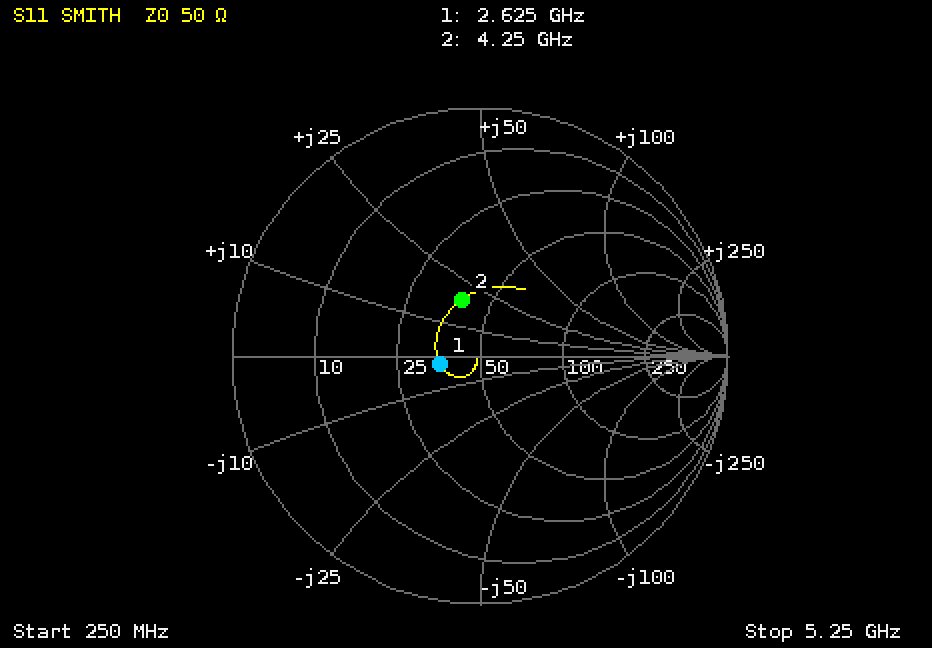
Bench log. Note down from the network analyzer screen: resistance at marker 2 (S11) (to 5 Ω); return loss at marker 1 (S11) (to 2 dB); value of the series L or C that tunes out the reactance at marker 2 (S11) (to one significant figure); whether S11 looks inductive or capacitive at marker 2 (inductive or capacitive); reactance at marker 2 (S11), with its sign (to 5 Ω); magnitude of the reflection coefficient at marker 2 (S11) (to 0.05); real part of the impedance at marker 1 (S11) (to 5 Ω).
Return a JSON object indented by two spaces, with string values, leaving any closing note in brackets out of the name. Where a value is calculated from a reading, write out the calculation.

{
  "resistance at marker 2 (S11)": "40 Ω",
  "return loss at marker 1 (S11)": "16 dB",
  "value of the series L or C that tunes out the reactance at marker 2 (S11)": "C = 1/(2π × 4.25 GHz × 20 Ω) ≈ 2 pF",
  "whether S11 looks inductive or capacitive at marker 2": "inductive",
  "reactance at marker 2 (S11), with its sign": "+20 Ω",
  "magnitude of the reflection coefficient at marker 2 (S11)": "0.25",
  "real part of the impedance at marker 1 (S11)": "35 Ω"
}
